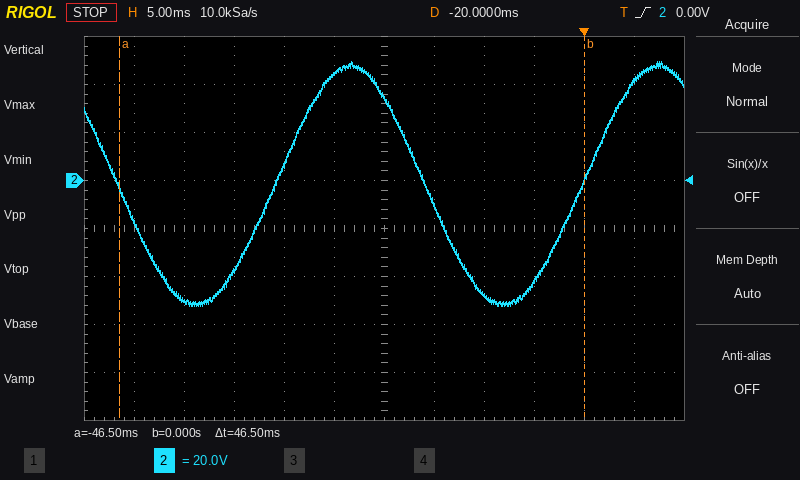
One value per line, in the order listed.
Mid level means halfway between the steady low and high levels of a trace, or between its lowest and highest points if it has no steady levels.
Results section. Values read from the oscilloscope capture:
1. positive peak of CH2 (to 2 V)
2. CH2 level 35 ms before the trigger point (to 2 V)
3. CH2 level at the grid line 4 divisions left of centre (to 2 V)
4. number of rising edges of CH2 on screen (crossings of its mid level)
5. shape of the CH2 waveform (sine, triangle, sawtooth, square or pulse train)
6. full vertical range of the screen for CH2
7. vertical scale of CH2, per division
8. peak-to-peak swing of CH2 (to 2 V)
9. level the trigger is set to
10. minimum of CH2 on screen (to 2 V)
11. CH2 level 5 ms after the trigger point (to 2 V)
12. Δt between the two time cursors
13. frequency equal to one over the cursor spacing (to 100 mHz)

50 V
-38 V
-50 V
2
sine
160 V
20 V
102 V
0.00 V
-52 V
42 V
46.5 ms
21.5 Hz
